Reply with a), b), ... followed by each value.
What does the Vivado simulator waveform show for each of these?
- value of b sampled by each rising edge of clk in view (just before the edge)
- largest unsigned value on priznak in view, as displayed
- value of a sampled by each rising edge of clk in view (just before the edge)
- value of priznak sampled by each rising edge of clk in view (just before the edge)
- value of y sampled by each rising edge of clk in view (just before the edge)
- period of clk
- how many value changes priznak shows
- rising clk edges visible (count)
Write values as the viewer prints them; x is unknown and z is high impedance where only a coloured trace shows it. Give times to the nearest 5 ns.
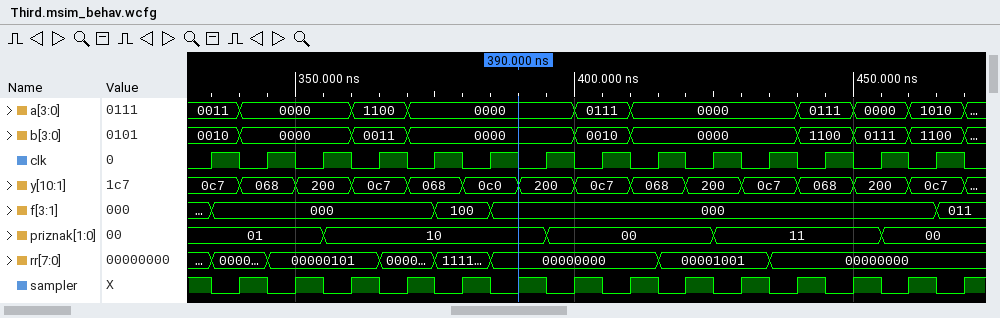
a) 0010, 0000, 0000, 0011, 0000, 0000, 0000, 0010, 0000, 0000, 0000, 1100, 0111, 1100
b) 11
c) 0011, 0000, 0000, 1100, 0000, 0000, 0000, 0111, 0000, 0000, 0000, 0111, 0000, 1010
d) 01, 01, 01, 10, 10, 10, 10, 00, 00, 00, 11, 11, 11, 00
e) 0c7, 068, 200, 0c7, 068, 0c0, 200, 0c7, 068, 200, 0c7, 068, 200, 0c7
f) 10 ns
g) 4
h) 14
